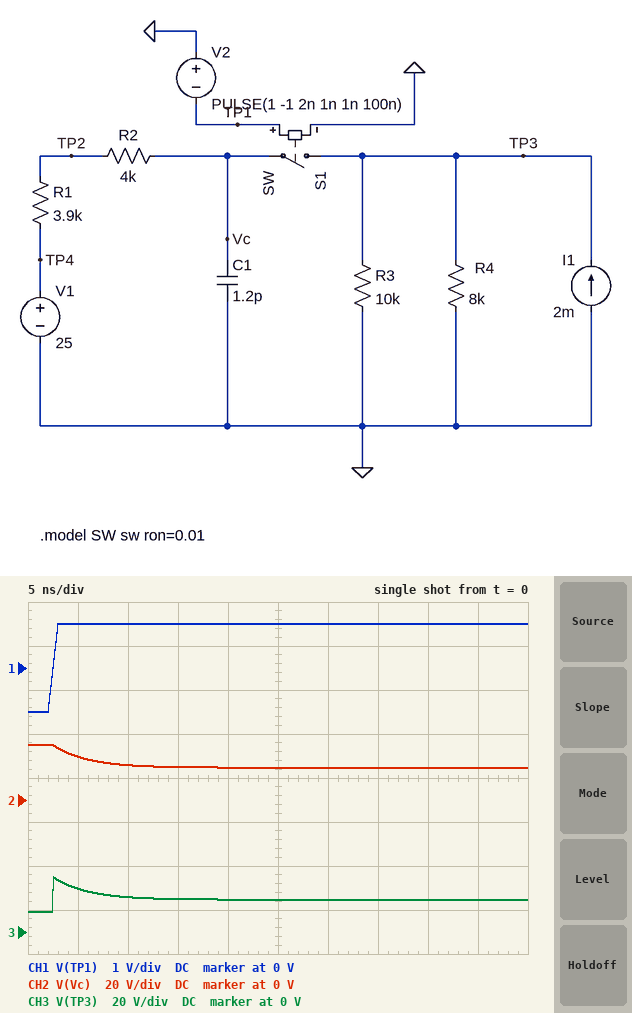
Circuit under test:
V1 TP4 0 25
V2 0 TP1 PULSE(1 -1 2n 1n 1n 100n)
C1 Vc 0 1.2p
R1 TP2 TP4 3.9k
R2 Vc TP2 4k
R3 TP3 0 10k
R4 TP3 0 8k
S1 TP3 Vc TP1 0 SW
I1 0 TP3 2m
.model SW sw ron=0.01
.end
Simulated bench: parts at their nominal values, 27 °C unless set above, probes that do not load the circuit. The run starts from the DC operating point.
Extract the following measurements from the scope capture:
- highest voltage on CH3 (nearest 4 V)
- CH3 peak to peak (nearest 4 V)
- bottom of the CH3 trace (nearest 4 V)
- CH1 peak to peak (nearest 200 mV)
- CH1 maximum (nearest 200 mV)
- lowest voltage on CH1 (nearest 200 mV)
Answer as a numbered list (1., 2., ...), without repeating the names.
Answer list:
1. 24 V
2. 16 V
3. 8 V
4. 2.0 V
5. 1.0 V
6. -1.0 V
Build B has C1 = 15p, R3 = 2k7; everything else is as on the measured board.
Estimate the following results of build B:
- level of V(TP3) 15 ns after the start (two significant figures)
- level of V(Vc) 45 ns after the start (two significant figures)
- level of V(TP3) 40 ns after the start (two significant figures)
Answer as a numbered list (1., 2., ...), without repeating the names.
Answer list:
1. 18 V
2. 11 V
3. 12 V
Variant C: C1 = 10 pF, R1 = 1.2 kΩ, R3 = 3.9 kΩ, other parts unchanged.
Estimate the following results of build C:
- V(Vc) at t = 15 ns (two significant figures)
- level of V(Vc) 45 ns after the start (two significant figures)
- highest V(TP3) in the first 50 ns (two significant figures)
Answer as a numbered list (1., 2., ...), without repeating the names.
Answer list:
1. 18 V
2. 13 V
3. 25 V
